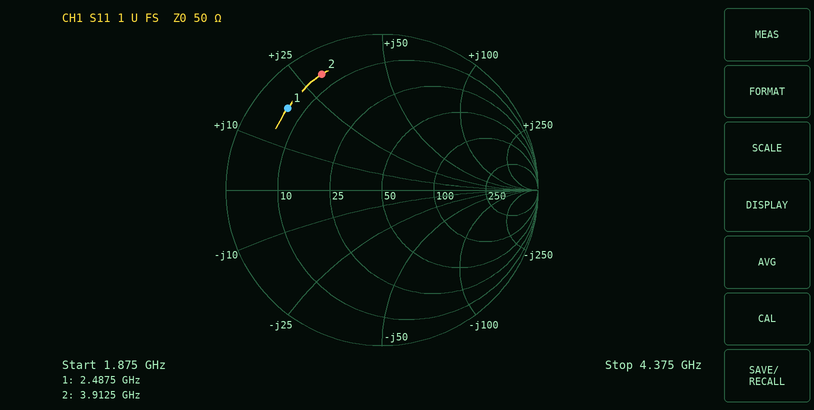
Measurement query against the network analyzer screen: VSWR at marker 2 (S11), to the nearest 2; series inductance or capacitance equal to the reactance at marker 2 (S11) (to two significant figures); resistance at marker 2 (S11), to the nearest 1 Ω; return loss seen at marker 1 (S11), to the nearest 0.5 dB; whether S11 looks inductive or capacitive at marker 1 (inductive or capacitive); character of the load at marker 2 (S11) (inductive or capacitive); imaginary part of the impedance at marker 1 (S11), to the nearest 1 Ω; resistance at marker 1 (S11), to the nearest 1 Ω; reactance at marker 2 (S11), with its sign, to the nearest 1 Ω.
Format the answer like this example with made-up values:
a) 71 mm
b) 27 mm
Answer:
a) 12
b) 1.2 nH
c) 6 Ω
d) 2.0 dB
e) inductive
f) inductive
g) +18 Ω
h) 6 Ω
i) +30 Ω
